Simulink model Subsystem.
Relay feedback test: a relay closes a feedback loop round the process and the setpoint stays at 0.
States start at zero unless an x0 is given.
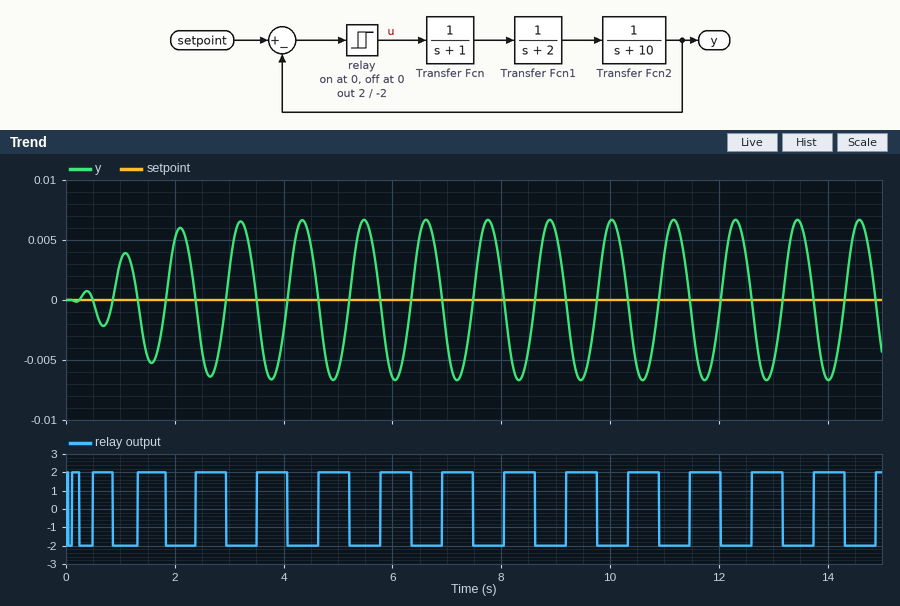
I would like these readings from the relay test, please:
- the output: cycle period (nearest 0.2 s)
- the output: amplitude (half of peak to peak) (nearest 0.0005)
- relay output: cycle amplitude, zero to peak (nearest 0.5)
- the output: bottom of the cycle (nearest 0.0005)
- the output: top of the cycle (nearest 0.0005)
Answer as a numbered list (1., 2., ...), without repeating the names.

1. 1.2 s
2. 0.0065
3. 2.0
4. -0.0065
5. 0.0065
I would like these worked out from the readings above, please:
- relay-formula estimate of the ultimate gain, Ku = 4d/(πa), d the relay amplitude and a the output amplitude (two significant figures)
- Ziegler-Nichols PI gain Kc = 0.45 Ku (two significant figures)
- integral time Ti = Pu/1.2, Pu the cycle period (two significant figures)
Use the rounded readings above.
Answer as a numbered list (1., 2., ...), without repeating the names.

1. 390
2. 180
3. 1.0 s
